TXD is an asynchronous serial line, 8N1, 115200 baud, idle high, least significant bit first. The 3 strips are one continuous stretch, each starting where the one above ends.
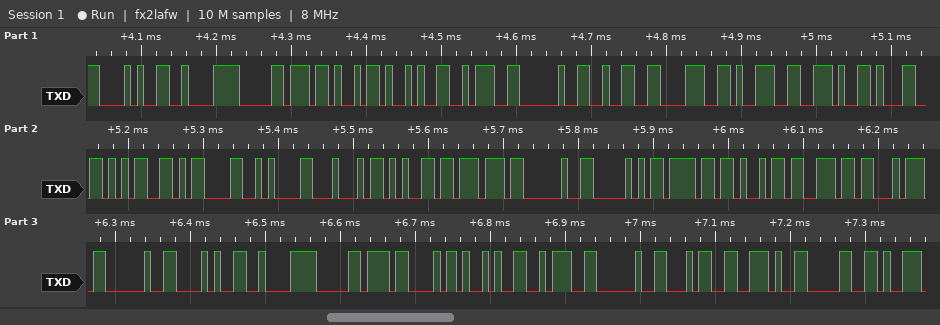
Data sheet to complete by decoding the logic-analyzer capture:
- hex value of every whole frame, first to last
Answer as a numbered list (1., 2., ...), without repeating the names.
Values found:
1. 28 C2 B0 4B 29 3A 20 32 38 39 2E 31 35 0D 0A 44 65 77 20 50 6F 69 6E 74 20 28 C2 B0 43 29 3A 20 34 2E 30
